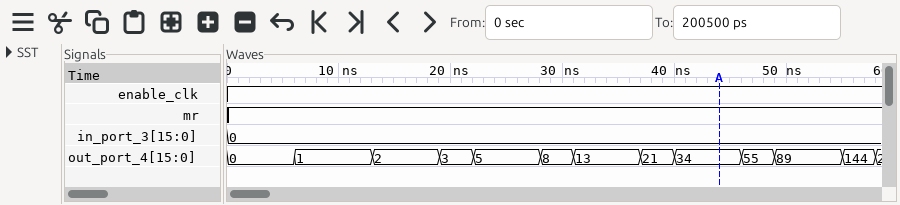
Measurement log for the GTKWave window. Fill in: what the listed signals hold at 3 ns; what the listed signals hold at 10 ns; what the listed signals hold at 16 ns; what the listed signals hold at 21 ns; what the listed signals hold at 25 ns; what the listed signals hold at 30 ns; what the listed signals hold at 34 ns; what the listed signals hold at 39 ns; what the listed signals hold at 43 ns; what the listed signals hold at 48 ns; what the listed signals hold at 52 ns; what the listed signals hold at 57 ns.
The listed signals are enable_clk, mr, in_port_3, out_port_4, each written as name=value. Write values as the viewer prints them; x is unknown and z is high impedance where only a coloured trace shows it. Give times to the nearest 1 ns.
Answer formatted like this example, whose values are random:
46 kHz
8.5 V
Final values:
enable_clk=1, mr=1, in_port_3=0, out_port_4=0
enable_clk=1, mr=1, in_port_3=0, out_port_4=1
enable_clk=1, mr=1, in_port_3=0, out_port_4=2
enable_clk=1, mr=1, in_port_3=0, out_port_4=3
enable_clk=1, mr=1, in_port_3=0, out_port_4=5
enable_clk=1, mr=1, in_port_3=0, out_port_4=8
enable_clk=1, mr=1, in_port_3=0, out_port_4=13
enable_clk=1, mr=1, in_port_3=0, out_port_4=21
enable_clk=1, mr=1, in_port_3=0, out_port_4=34
enable_clk=1, mr=1, in_port_3=0, out_port_4=55
enable_clk=1, mr=1, in_port_3=0, out_port_4=89
enable_clk=1, mr=1, in_port_3=0, out_port_4=144
